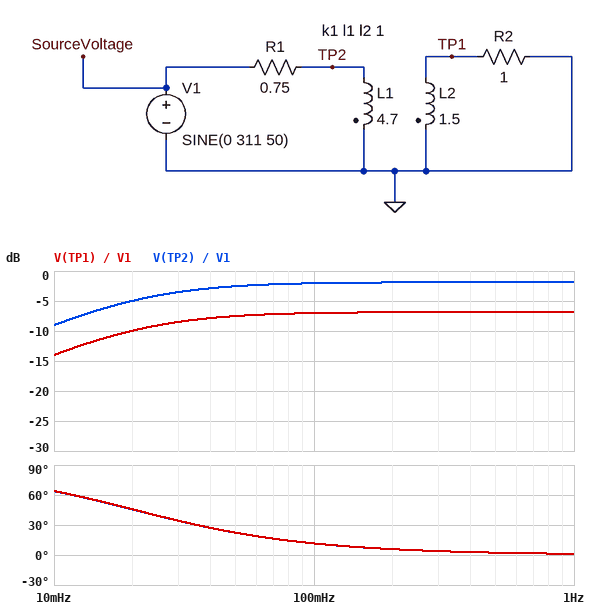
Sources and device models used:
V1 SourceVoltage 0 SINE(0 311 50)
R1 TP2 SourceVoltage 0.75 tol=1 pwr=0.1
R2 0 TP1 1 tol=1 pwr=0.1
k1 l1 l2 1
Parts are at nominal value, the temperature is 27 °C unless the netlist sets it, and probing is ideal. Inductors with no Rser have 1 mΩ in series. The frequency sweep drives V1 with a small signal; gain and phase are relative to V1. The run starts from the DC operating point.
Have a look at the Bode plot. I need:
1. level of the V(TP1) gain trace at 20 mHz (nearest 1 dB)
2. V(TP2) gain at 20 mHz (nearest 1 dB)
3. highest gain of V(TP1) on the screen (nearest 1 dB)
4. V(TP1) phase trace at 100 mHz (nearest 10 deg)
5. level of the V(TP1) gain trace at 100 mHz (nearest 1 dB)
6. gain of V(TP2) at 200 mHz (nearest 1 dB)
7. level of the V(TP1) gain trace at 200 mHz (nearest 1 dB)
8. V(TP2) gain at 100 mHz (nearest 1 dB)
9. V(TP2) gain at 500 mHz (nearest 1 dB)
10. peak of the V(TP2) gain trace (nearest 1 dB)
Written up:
-10 dB
-5 dB
-7 dB
10 deg
-7 dB
-2 dB
-7 dB
-2 dB
-2 dB
-2 dB
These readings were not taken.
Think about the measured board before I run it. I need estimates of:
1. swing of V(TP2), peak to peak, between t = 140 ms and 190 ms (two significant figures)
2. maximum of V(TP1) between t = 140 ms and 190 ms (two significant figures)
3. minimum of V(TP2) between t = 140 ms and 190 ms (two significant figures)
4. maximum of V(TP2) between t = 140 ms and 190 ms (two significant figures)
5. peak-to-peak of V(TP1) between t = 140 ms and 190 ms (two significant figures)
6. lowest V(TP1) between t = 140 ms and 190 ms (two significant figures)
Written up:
500 V
140 V
-250 V
250 V
280 V
-140 V
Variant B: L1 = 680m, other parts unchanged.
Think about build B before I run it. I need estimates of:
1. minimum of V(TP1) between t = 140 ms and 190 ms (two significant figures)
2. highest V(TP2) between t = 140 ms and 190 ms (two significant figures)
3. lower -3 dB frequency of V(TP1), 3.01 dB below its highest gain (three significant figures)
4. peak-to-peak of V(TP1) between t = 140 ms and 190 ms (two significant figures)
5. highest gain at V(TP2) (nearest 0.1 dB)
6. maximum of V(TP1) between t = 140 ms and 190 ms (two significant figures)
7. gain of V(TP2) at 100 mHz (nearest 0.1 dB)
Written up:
-170 V
120 V
66.2 mHz
350 V
-8.5 dB
170 V
-10.0 dB
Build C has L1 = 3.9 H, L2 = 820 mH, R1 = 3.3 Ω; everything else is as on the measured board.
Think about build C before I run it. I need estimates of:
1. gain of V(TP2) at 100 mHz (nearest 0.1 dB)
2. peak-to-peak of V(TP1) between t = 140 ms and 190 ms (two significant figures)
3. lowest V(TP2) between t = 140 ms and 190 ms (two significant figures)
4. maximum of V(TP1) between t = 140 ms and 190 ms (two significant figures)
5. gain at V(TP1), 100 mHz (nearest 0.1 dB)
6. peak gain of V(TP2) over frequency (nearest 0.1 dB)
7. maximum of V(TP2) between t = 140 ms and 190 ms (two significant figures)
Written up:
-6.7 dB
170 V
-180 V
84 V
-13.5 dB
-4.6 dB
180 V
